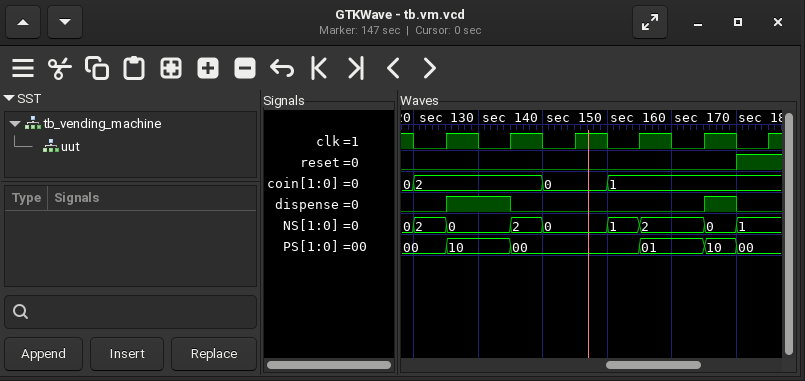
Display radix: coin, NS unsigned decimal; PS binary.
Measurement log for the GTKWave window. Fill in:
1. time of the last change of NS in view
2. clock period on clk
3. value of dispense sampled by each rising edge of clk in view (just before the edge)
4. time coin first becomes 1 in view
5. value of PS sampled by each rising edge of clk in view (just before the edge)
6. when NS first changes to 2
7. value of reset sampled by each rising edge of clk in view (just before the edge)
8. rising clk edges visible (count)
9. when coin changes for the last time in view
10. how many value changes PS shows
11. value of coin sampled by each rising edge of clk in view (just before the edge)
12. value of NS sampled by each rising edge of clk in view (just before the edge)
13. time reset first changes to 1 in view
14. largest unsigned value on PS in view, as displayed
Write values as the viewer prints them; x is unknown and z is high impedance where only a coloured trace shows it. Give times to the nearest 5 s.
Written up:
170 s
10 s
0 1 0 0 0 0
150 s
00, 10, 00, 00, 01, 00
120 s
0 0 0 0 0 1
6
150 s
5
2, 2, 0, 1, 1, 1
2, 0, 0, 1, 2, 1
170 s
10
